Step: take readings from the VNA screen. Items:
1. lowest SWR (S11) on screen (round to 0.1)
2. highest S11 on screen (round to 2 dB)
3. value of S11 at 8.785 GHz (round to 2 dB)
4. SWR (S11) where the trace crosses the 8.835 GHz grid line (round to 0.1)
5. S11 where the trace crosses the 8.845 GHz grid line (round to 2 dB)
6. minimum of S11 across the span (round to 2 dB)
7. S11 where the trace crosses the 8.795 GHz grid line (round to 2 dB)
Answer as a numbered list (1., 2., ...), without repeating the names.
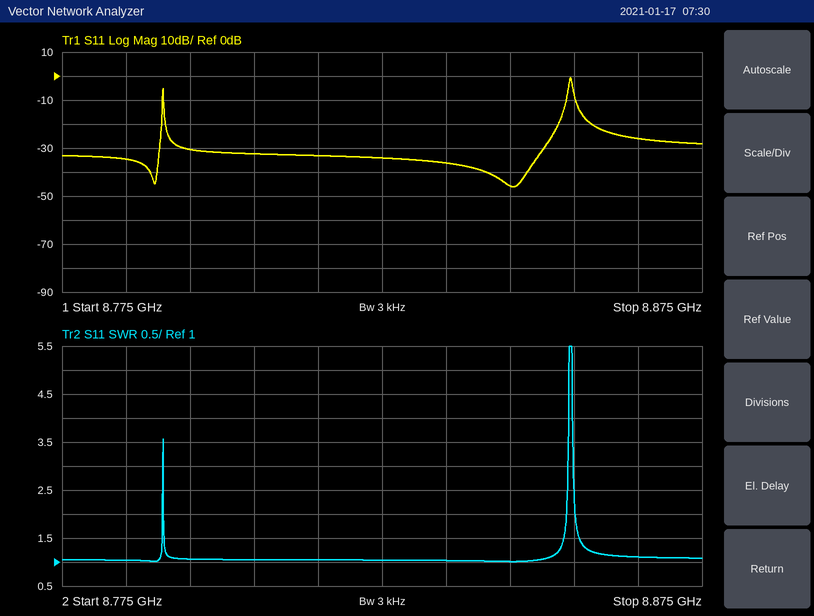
1. 1.0
2. 0 dB
3. -34 dB
4. 1.0
5. -46 dB
6. -46 dB
7. -30 dB
